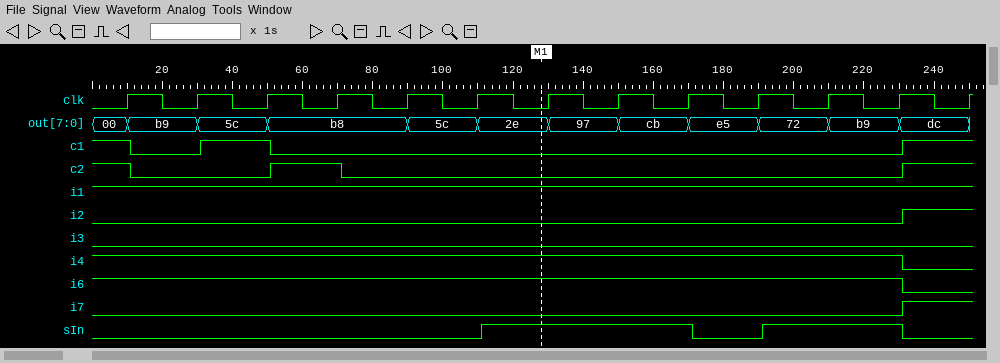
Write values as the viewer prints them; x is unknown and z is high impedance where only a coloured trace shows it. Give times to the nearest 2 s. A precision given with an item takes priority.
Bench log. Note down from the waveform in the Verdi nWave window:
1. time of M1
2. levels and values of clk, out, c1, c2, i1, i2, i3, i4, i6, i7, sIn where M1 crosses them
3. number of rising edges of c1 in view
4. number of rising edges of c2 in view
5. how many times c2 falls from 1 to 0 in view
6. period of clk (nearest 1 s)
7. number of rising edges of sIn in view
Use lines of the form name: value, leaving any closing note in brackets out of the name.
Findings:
time of M1: 128 s
levels and values of clk, out, c1, c2, i1, i2, i3, i4, i6, i7, sIn where M1 crosses them: clk=0, out=2e, c1=0, c2=0, i1=1, i2=0, i3=0, i4=1, i6=1, i7=0, sIn=1
number of rising edges of c1 in view: 2
number of rising edges of c2 in view: 2
how many times c2 falls from 1 to 0 in view: 2
period of clk: 20 s
number of rising edges of sIn in view: 2
